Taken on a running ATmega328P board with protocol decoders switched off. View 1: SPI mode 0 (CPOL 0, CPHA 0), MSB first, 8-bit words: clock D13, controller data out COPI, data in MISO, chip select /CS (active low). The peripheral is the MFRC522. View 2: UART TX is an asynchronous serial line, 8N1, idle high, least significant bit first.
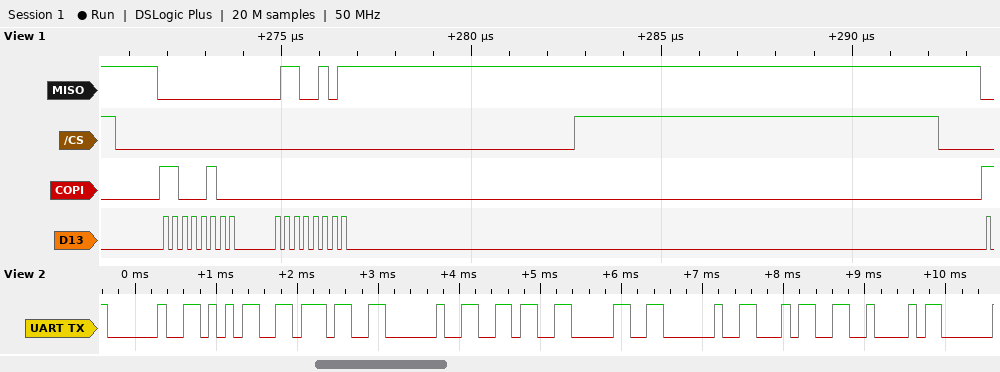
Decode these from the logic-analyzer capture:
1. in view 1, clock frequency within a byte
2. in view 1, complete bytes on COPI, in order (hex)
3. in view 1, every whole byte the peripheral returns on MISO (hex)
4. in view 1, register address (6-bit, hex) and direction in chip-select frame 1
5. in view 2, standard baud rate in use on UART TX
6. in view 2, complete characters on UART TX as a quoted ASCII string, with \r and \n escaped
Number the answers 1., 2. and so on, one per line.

1. 4 MHz
2. C4 00
3. 00 65
4. 0x22 read
5. 9600 baud
6. " 57 60 4B"
